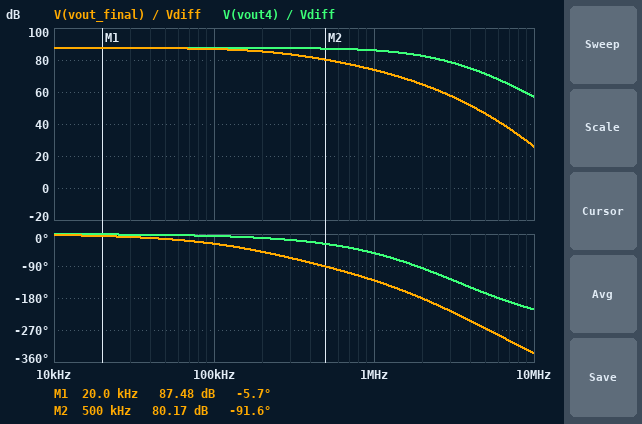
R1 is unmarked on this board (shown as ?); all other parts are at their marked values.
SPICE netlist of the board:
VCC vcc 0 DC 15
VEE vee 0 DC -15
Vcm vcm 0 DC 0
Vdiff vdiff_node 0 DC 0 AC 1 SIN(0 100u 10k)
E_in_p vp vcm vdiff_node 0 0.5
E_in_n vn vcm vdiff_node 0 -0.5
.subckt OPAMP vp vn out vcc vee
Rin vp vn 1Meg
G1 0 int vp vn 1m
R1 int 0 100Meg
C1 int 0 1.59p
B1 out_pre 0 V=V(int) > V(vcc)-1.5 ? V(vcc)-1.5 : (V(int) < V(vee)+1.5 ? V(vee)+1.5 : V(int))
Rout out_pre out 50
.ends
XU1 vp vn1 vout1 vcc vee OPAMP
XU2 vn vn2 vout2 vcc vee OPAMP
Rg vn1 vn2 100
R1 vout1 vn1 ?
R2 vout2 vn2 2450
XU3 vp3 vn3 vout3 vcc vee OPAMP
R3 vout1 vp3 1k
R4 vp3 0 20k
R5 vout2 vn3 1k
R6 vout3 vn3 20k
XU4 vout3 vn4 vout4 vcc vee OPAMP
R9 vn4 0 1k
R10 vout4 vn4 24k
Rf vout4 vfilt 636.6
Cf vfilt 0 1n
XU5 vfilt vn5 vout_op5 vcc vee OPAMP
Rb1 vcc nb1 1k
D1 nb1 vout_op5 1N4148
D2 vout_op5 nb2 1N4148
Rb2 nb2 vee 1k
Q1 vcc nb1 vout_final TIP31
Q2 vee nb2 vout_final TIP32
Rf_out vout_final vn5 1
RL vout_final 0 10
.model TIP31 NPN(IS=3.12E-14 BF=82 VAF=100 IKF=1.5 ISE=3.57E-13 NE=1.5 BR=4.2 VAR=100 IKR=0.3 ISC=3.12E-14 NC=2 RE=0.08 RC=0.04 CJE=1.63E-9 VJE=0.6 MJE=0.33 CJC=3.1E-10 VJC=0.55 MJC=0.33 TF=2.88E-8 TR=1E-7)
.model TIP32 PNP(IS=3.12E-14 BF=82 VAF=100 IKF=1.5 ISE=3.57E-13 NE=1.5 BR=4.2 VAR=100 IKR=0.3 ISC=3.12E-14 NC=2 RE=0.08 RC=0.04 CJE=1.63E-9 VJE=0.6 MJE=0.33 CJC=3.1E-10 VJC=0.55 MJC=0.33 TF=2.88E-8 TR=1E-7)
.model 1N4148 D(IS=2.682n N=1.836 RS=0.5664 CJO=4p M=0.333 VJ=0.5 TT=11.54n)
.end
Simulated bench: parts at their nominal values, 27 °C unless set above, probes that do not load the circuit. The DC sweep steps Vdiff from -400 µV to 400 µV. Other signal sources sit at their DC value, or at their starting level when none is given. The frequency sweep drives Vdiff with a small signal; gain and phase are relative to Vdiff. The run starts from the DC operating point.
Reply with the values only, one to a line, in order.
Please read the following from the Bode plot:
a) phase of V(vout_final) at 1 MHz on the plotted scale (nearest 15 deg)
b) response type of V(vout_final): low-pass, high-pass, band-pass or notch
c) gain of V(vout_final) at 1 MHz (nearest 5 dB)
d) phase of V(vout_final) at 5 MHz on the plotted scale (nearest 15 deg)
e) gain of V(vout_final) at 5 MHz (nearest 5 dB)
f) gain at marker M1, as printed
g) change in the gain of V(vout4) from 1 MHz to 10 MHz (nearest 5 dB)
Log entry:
-135 deg
low-pass
75 dB
-270 deg
45 dB
87.48 dB
-30 dB
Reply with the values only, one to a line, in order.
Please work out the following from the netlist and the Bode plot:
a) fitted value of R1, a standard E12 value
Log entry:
2.2 kΩ
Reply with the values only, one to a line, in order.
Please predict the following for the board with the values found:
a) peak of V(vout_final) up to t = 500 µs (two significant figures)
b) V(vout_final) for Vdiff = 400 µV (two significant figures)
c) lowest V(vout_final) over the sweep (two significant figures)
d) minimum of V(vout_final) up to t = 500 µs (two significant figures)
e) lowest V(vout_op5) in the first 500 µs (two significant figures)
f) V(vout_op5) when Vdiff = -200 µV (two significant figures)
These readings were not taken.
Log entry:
2.4 V
5.6 V
-5.6 V
-2.4 V
-2.4 V
-4.9 V
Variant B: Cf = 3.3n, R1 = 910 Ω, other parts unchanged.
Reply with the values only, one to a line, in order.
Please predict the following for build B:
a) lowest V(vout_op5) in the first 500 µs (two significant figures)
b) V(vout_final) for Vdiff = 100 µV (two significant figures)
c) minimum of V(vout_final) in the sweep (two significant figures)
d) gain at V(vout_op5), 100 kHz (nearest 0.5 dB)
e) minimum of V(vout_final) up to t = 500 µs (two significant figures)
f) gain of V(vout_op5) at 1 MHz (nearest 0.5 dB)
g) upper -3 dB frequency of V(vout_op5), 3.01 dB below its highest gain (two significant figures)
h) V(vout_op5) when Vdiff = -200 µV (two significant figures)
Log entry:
-1.8 V
1.7 V
-5.6 V
80.5 dB
-1.7 V
61.5 dB
76 kHz
-3.6 V
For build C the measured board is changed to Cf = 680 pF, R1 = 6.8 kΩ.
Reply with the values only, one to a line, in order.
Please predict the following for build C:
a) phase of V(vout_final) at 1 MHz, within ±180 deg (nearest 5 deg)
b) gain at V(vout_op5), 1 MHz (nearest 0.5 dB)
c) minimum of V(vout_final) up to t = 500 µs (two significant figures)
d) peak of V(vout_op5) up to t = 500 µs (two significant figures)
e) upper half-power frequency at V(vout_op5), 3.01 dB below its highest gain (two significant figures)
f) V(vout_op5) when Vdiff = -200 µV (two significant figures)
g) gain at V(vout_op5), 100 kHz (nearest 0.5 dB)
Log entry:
-140 deg
81.0 dB
-4.7 V
4.8 V
330 kHz
-12 V
93.5 dB
